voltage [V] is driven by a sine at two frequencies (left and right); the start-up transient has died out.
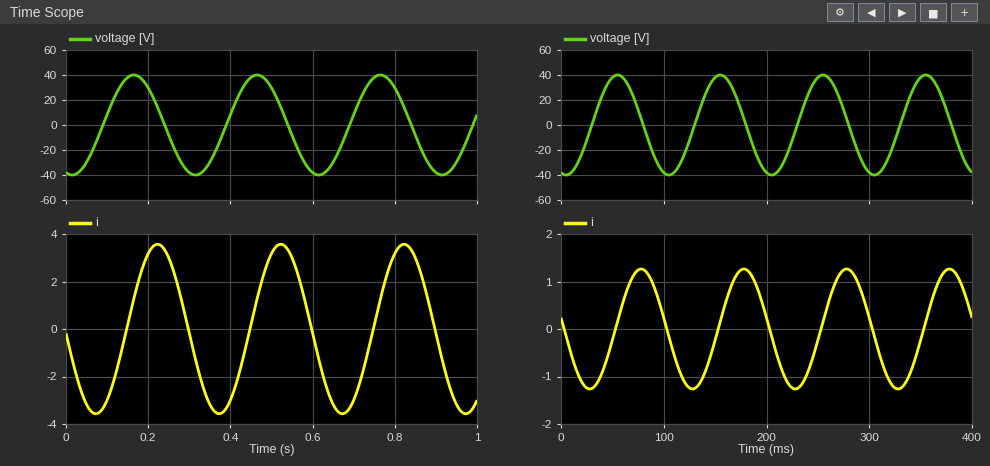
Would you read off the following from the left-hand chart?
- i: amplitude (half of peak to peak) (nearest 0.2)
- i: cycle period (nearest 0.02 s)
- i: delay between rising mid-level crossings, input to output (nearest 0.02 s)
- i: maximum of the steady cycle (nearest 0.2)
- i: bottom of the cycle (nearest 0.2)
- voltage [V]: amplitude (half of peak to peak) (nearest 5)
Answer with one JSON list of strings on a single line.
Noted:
["3.6", "0.30 s", "0.06 s", "3.6", "-3.6", "40"]
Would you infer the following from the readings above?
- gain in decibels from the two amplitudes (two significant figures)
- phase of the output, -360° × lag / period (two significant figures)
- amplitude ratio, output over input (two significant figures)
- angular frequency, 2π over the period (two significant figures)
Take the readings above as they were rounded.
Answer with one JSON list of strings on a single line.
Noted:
["-21 dB", "-72°", "0.090", "21 rad/s"]
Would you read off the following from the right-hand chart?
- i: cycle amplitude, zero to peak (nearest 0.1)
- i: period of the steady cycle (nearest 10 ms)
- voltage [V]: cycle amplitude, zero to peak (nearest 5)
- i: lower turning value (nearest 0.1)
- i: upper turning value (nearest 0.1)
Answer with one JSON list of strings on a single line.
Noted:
["1.3", "100 ms", "40", "-1.3", "1.3"]
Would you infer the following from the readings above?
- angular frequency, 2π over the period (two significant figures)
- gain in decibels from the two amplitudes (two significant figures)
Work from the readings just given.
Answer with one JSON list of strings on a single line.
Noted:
["0.063 rad/ms", "-30 dB"]
